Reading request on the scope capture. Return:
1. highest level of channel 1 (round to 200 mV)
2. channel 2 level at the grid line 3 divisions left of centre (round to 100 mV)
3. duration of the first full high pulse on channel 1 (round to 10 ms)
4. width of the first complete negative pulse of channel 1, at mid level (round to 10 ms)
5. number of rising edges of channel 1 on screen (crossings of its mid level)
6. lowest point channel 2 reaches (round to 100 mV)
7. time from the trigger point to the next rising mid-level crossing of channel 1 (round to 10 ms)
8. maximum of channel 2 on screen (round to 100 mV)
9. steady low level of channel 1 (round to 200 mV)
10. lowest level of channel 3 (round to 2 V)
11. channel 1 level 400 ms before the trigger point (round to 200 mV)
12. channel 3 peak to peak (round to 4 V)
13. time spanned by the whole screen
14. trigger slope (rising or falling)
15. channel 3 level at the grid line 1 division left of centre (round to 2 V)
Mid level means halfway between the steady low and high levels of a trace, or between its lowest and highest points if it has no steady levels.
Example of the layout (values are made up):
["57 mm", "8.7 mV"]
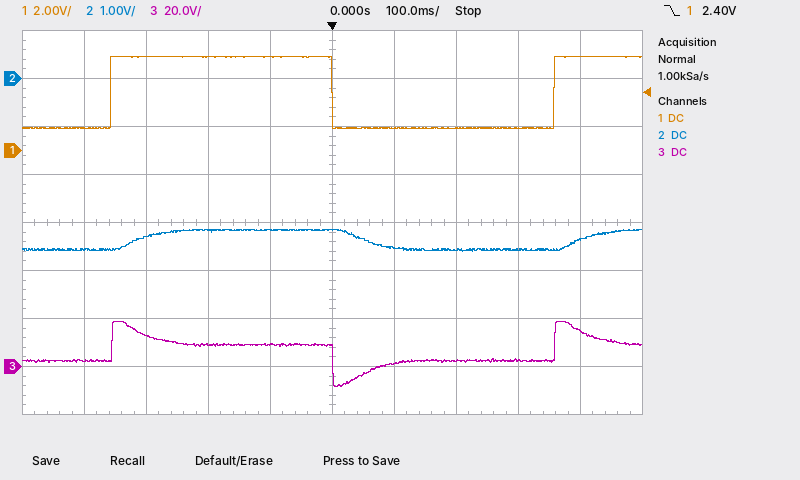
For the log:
["4.0 V", "-3.3 V", "360 ms", "360 ms", "2", "-3.6 V", "360 ms", "-3.1 V", "1.0 V", "-8 V", "1.0 V", "28 V", "1 s", "falling", "10 V"]
